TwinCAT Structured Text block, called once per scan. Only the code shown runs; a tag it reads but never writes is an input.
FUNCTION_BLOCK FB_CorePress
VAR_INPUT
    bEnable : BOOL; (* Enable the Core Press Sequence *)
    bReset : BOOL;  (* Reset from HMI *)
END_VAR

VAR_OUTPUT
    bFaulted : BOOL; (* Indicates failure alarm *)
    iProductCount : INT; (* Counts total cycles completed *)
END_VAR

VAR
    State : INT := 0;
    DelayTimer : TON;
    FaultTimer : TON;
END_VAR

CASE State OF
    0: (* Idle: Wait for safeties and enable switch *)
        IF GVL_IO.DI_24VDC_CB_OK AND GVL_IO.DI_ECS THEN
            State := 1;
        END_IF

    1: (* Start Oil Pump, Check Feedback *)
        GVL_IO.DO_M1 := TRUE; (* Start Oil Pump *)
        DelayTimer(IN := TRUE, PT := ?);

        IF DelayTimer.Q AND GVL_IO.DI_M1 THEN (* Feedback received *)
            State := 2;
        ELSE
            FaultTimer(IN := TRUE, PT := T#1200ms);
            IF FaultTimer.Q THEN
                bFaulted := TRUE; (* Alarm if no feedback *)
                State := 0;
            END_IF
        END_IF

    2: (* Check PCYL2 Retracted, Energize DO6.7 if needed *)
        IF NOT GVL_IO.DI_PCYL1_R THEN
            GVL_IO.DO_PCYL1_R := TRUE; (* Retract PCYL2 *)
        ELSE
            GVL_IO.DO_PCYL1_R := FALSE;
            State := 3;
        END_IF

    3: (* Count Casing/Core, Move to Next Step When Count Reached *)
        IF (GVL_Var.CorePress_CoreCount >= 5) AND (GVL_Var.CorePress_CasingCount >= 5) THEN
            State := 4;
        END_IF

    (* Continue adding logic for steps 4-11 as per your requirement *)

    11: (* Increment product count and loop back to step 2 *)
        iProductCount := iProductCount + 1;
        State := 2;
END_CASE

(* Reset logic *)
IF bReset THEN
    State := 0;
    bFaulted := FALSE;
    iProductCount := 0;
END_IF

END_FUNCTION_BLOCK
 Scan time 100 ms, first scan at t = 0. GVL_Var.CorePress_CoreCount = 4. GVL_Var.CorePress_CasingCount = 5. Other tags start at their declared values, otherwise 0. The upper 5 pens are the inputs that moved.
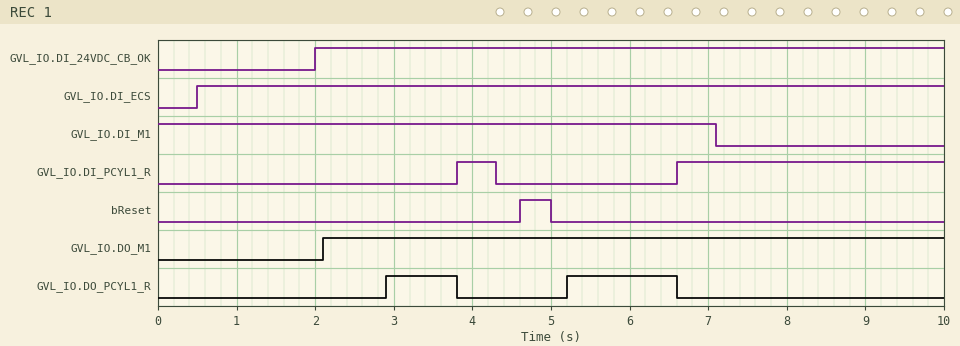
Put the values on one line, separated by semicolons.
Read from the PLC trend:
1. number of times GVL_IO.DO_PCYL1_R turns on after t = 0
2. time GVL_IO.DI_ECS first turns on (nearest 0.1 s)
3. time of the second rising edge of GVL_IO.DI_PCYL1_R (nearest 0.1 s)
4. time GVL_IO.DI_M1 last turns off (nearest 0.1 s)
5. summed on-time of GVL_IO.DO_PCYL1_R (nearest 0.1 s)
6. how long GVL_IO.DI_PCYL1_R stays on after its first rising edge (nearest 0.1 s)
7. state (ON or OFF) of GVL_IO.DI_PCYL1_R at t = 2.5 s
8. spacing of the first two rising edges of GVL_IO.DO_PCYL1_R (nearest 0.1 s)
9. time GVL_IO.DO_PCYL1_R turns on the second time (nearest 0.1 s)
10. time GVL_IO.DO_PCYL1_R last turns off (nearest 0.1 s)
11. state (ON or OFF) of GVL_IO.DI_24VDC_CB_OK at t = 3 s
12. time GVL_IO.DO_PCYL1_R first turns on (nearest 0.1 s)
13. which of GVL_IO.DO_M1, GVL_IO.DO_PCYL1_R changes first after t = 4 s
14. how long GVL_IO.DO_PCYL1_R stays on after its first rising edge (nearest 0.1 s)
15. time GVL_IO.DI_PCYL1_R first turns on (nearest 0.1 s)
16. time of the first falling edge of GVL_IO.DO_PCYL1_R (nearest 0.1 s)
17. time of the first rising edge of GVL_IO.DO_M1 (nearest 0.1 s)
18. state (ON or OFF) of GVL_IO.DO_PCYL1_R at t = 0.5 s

2; 0.5 s; 6.6 s; 7.1 s; 2.3 s; 0.5 s; OFF; 2.3 s; 5.2 s; 6.6 s; ON; 2.9 s; GVL_IO.DO_PCYL1_R; 0.9 s; 3.8 s; 3.8 s; 2.1 s; OFF
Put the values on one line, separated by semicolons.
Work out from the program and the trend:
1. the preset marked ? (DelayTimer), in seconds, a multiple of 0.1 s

0.7 s
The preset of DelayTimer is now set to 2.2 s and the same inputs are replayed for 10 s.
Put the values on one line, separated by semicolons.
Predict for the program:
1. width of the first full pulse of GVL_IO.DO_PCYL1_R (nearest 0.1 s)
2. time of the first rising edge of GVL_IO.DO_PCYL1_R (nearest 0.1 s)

2.2 s; 4.4 s
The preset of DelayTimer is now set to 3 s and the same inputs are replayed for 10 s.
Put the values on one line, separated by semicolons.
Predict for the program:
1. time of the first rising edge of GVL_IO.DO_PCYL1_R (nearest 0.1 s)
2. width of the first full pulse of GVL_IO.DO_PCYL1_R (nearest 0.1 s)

5.2 s; 1.4 s
